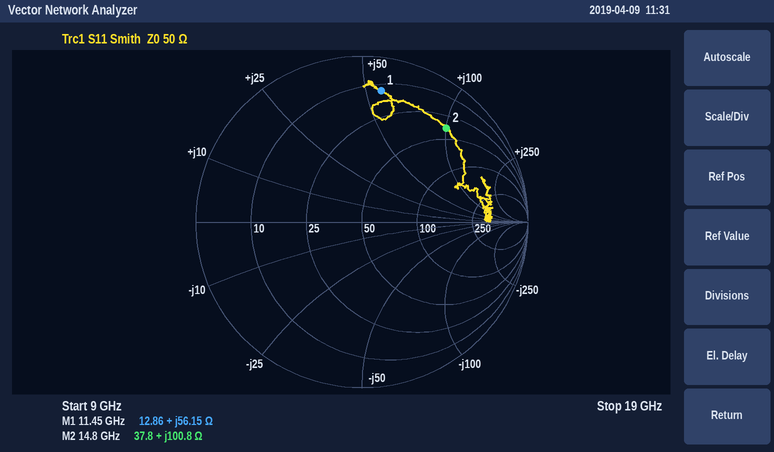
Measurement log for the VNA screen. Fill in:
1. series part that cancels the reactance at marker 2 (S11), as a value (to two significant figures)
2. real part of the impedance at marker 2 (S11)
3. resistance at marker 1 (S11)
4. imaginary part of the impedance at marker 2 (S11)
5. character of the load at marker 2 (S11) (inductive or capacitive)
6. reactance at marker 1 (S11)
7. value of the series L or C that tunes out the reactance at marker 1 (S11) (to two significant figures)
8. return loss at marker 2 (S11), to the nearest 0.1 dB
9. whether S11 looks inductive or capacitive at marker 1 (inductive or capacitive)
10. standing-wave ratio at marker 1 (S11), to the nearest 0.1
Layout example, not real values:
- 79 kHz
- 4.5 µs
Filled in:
- 110 fF
- 37.8 Ω
- 12.86 Ω
- +100.8 Ω
- inductive
- +56.15 Ω
- 250 fF
- 2.4 dB
- inductive
- 8.9
